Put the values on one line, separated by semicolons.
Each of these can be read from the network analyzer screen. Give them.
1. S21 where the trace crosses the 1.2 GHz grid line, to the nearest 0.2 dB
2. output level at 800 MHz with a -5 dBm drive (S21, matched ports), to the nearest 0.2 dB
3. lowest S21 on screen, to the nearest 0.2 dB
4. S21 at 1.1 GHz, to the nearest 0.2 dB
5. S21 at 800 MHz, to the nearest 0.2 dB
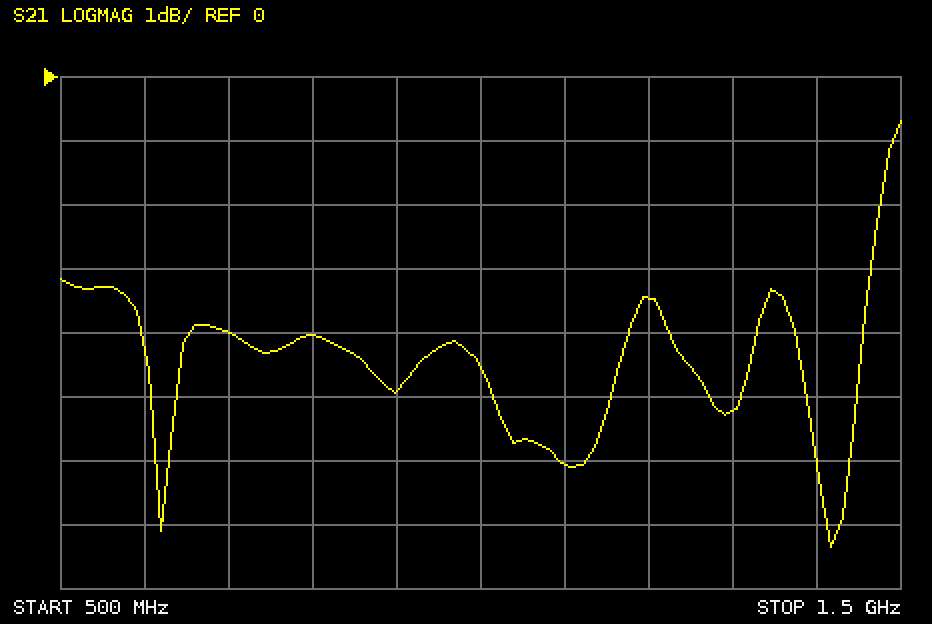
-3.4 dB; -9.0 dBm; -7.4 dB; -6.0 dB; -4.0 dB
